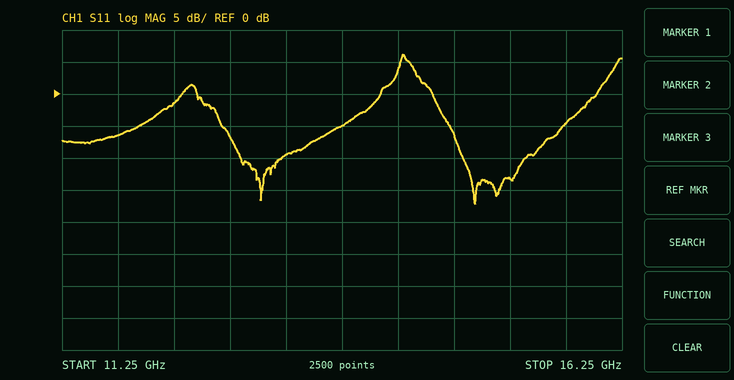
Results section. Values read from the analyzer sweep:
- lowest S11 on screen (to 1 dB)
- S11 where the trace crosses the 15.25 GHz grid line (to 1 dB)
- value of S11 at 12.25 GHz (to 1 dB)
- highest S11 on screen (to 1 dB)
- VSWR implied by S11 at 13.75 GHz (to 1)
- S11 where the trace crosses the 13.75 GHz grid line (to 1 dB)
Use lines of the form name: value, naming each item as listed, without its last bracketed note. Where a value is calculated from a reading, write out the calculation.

lowest S11 on screen: -17 dB
S11 where the trace crosses the 15.25 GHz grid line: -13 dB
value of S11 at 12.25 GHz: -1 dB
highest S11 on screen: 6 dB
VSWR implied by S11 at 13.75 GHz: |Γ| = 10^(-5/20) = 0.5623; VSWR = (1 + 0.5623)/(1 − 0.5623) ≈ 4
S11 where the trace crosses the 13.75 GHz grid line: -5 dB
